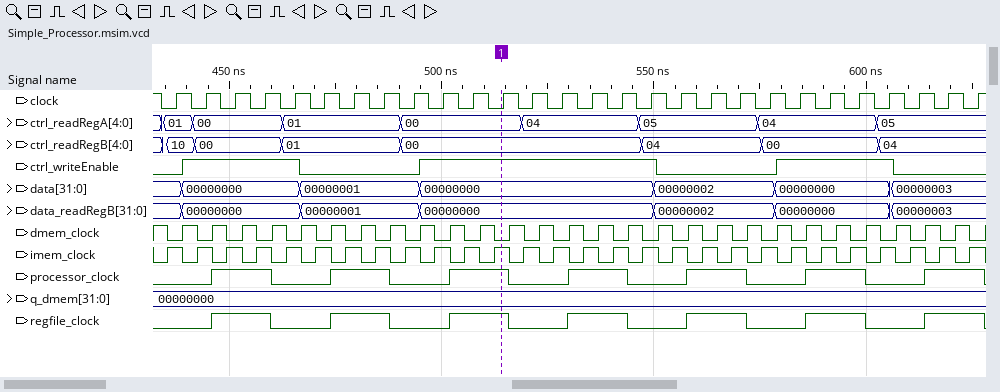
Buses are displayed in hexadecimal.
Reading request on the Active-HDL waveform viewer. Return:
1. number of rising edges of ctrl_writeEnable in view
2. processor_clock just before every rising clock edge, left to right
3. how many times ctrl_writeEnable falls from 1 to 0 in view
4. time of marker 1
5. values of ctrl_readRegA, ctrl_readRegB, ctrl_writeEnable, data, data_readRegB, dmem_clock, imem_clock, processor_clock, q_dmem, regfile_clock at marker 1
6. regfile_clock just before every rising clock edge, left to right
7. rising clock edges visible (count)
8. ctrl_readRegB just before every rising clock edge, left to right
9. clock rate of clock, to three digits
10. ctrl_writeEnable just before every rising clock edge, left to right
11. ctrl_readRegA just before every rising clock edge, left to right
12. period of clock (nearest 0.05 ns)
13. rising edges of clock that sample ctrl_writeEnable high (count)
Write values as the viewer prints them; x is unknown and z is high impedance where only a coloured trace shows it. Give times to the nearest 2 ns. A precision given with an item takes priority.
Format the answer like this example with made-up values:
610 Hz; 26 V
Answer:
3; 0 0 1 1 0 0 1 1 0 0 1 1 0 0 1 1 0 0 1 1 0 0 1 1 0 0 1 1; 3; 514 ns; ctrl_readRegA=00, ctrl_readRegB=00, ctrl_writeEnable=1, data=00000000, data_readRegB=00000000, dmem_clock=0, imem_clock=1, processor_clock=1, q_dmem=00000000, regfile_clock=1; 0 0 1 1 0 0 1 1 0 0 1 1 0 0 1 1 0 0 1 1 0 0 1 1 0 0 1 1; 28; 10, 00, 00, 00, 01, 01, 01, 01, 00, 00, 00, 00, 00, 00, 00, 00, 04, 04, 04, 04, 00, 00, 00, 00, 04, 04, 04, 04; 143 MHz; 0 1 1 1 1 0 0 0 0 1 1 1 1 1 1 1 1 0 0 0 0 1 1 1 1 0 0 0; 01, 00, 00, 00, 01, 01, 01, 01, 00, 00, 00, 00, 04, 04, 04, 04, 05, 05, 05, 05, 04, 04, 04, 04, 05, 05, 05, 05; 7 ns; 16
